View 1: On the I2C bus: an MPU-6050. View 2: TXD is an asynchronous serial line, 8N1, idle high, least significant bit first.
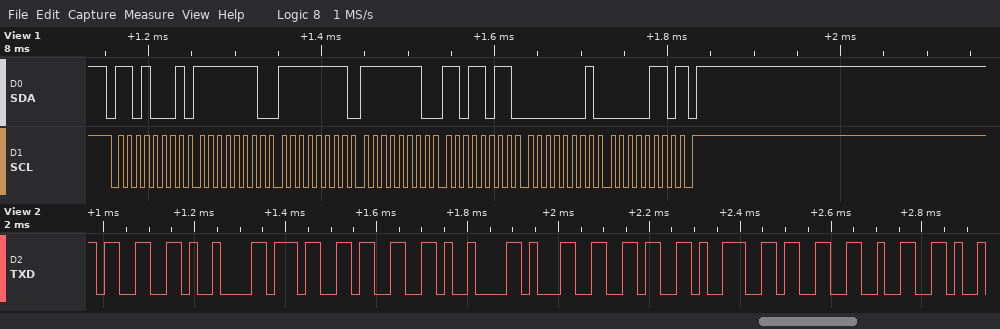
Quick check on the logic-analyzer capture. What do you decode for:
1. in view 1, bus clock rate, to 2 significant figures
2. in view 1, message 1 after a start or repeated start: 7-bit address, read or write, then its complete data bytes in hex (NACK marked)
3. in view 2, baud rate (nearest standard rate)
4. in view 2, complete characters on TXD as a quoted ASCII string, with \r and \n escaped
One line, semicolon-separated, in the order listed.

100 kHz; 0x68 read: FE FF FE DB 01 06 NACK; 57600 baud; "3\t73\t16932"
